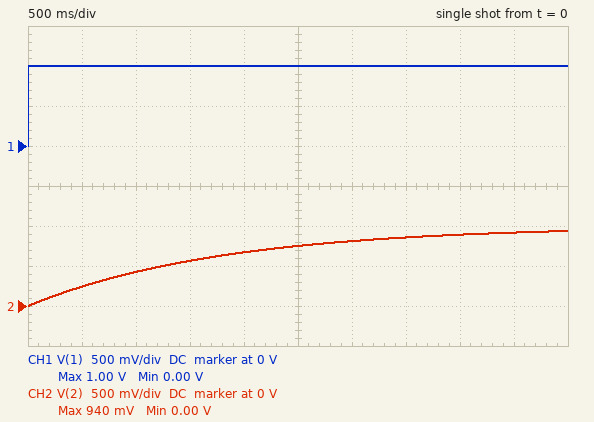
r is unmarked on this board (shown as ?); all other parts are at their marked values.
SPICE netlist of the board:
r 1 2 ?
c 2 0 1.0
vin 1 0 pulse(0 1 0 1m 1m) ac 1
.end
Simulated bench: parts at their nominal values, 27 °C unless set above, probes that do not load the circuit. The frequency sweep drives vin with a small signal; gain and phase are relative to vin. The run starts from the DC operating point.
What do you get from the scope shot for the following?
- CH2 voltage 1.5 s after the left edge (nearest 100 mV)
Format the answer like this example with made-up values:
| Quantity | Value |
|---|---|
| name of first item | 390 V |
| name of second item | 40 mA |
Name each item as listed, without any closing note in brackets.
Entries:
| Quantity | Value |
|---|---|
| CH2 voltage 1.5 s after the left edge | 600 mV |
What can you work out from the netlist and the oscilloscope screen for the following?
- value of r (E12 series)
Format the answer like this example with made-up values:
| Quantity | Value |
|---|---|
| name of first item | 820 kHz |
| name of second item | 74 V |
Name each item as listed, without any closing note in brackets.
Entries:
| Quantity | Value |
|---|---|
| value of r | 1.8 Ω |
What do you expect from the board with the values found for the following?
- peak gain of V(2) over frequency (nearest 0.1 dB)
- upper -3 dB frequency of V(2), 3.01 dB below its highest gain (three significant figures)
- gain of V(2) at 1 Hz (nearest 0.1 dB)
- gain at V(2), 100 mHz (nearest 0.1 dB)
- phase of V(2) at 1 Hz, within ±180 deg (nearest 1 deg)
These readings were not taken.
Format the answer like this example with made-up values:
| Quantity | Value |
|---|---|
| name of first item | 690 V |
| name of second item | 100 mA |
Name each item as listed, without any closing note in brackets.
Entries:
| Quantity | Value |
|---|---|
| peak gain of V(2) over frequency | 0 dB |
| upper -3 dB frequency of V(2), 3.01 dB below its highest gain | 88.4 mHz |
| gain of V(2) at 1 Hz | -21.1 dB |
| gain at V(2), 100 mHz | -3.6 dB |
| phase of V(2) at 1 Hz, within ±180 deg | -85 deg |
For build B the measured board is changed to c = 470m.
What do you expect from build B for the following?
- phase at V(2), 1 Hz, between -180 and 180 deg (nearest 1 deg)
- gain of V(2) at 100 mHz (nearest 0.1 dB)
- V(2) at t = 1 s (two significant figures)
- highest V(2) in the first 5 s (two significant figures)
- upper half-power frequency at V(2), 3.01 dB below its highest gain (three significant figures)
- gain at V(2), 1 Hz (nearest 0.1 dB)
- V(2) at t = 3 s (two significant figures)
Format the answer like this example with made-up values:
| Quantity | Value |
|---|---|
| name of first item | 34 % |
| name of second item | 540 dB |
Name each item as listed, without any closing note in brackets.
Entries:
| Quantity | Value |
|---|---|
| phase at V(2), 1 Hz, between -180 and 180 deg | -79 deg |
| gain of V(2) at 100 mHz | -1.1 dB |
| V(2) at t = 1 s | 690 mV |
| highest V(2) in the first 5 s | 1.0 V |
| upper half-power frequency at V(2), 3.01 dB below its highest gain | 188 mHz |
| gain at V(2), 1 Hz | -14.7 dB |
| V(2) at t = 3 s | 970 mV |
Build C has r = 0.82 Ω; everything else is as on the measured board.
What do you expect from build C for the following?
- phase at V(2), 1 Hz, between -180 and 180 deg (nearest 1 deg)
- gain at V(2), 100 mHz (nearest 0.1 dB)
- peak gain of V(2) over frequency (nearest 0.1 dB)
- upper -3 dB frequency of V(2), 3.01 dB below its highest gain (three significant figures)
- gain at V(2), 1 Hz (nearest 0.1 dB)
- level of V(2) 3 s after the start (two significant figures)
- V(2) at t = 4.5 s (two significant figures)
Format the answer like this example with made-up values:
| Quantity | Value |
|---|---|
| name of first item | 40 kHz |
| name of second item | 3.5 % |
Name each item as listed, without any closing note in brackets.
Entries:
| Quantity | Value |
|---|---|
| phase at V(2), 1 Hz, between -180 and 180 deg | -79 deg |
| gain at V(2), 100 mHz | -1.0 dB |
| peak gain of V(2) over frequency | 0 dB |
| upper -3 dB frequency of V(2), 3.01 dB below its highest gain | 194 mHz |
| gain at V(2), 1 Hz | -14.4 dB |
| level of V(2) 3 s after the start | 970 mV |
| V(2) at t = 4.5 s | 1.0 V |
